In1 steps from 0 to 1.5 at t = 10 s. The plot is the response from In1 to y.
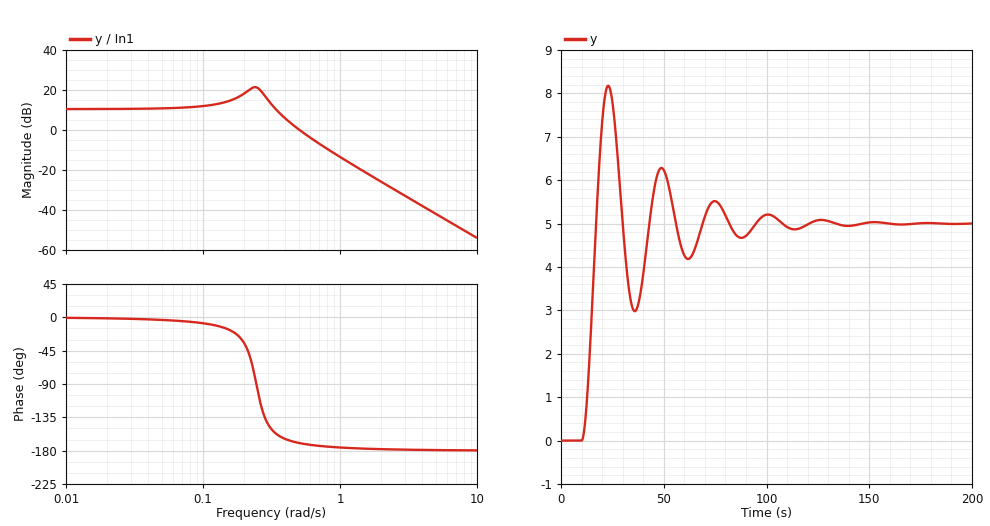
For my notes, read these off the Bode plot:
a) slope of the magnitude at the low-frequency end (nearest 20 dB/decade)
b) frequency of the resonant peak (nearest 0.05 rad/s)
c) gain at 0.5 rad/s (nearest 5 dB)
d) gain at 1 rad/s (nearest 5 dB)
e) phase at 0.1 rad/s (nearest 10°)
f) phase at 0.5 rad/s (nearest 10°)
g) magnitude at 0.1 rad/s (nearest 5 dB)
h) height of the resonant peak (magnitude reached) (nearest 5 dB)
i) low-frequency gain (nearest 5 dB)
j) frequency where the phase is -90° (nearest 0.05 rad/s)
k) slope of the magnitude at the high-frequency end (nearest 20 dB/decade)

0 dB/decade
0.25 rad/s
0 dB
-15 dB
-10°
-170°
10 dB
20 dB
10 dB
0.25 rad/s
-40 dB/decade
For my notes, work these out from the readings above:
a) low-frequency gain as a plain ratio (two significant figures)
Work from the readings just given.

3.2
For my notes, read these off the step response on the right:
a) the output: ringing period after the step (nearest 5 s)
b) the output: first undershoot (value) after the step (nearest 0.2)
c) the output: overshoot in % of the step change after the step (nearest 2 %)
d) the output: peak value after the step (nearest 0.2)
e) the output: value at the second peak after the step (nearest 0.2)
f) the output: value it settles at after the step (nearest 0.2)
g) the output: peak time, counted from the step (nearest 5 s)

25 s
3.0
64 %
8.2
6.2
5.0
15 s
